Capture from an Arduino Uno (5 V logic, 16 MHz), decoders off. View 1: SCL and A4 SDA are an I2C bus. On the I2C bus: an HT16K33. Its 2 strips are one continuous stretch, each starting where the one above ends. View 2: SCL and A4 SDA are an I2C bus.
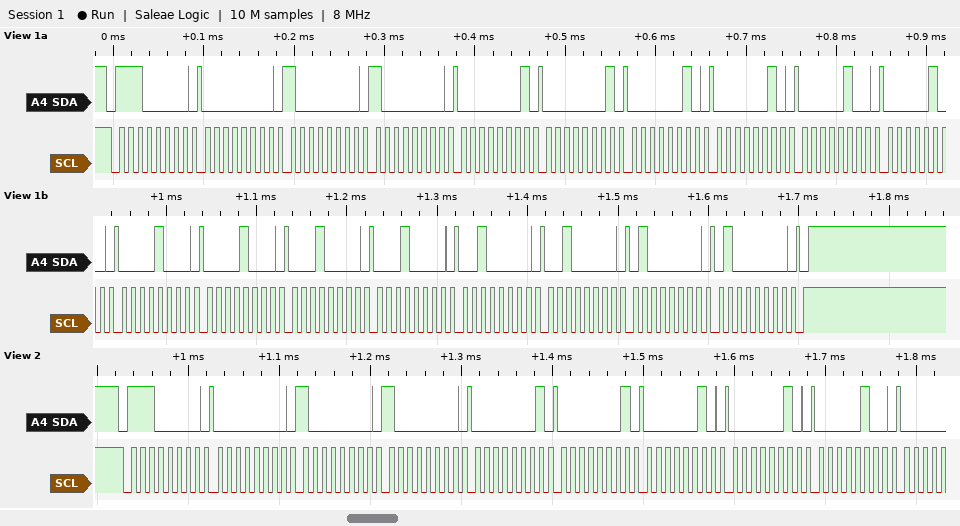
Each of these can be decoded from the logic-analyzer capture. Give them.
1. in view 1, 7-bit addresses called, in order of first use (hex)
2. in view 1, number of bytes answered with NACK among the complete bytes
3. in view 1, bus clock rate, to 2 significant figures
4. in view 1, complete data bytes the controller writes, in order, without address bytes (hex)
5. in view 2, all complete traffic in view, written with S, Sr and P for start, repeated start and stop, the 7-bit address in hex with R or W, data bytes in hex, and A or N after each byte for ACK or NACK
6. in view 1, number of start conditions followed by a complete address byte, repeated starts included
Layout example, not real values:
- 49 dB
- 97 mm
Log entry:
- 0x70
- 0
- 100 kHz
- 00 80 80 01 01 02 02 04 04 08 08 10 10 20 20 40 40
- S 70W A 00 A 80 A 80 A 01 A 01 A 02 A 02 A 04 A
- 1
